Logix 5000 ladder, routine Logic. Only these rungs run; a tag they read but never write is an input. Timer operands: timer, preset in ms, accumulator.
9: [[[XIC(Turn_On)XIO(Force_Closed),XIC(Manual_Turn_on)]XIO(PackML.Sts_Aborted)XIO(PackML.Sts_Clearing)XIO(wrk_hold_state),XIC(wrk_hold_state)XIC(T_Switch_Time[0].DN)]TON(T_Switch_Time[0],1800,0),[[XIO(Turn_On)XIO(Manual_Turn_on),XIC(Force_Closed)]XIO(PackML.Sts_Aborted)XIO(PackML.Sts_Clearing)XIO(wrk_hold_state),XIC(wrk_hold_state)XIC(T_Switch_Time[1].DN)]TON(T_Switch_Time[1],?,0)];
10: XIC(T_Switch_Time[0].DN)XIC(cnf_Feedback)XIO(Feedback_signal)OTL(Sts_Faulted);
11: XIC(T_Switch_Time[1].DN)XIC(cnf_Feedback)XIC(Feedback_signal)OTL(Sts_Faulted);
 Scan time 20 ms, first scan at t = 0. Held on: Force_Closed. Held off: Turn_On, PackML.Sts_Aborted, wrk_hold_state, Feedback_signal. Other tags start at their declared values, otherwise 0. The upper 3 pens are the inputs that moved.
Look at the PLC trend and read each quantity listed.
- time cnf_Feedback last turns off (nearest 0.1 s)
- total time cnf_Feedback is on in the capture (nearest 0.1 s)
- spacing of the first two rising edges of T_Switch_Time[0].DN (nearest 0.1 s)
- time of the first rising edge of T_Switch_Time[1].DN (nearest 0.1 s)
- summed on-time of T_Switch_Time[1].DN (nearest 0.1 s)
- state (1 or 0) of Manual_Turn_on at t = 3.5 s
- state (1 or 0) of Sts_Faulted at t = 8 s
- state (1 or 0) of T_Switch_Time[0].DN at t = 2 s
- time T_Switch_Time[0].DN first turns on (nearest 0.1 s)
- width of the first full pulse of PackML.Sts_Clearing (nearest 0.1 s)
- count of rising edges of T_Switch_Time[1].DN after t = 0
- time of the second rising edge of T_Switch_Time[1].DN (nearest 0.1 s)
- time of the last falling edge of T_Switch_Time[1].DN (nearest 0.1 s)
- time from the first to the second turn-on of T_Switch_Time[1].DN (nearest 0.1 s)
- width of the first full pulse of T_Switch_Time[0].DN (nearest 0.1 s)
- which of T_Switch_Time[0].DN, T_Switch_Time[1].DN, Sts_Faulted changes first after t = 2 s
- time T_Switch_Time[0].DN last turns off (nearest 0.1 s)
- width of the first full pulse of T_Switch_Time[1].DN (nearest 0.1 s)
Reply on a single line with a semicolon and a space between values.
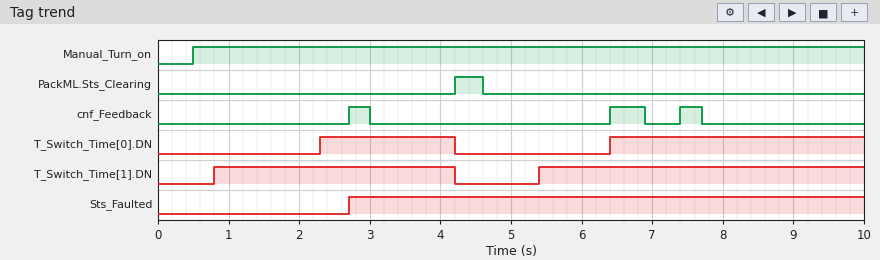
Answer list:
7.7 s; 1.1 s; 4.1 s; 0.8 s; 8.0 s; 1; 1; 0; 2.3 s; 0.4 s; 2; 5.4 s; 4.2 s; 4.6 s; 1.9 s; T_Switch_Time[0].DN; 4.2 s; 3.4 s
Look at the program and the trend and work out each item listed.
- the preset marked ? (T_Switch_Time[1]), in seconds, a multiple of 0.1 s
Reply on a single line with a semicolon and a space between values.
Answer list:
0.8 s
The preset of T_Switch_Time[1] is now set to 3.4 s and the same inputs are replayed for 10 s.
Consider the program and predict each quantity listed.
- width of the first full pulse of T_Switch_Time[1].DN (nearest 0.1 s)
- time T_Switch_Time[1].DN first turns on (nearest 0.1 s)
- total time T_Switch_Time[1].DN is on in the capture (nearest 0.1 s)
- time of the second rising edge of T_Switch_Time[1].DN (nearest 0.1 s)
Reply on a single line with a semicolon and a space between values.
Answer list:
0.8 s; 3.4 s; 2.8 s; 8.0 s
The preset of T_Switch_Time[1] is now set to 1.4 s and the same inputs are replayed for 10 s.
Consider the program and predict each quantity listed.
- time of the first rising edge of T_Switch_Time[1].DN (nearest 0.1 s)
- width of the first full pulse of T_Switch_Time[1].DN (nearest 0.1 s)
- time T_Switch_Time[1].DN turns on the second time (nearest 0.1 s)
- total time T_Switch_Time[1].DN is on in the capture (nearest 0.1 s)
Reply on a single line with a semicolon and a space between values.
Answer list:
1.4 s; 2.8 s; 6.0 s; 6.8 s
